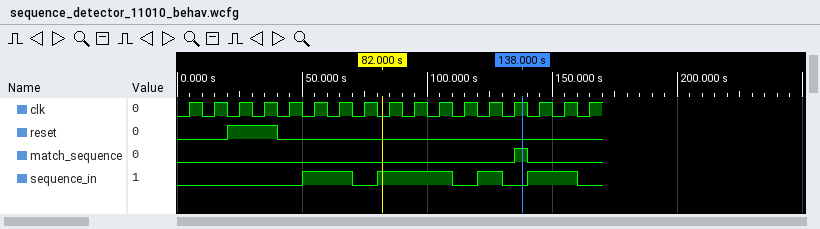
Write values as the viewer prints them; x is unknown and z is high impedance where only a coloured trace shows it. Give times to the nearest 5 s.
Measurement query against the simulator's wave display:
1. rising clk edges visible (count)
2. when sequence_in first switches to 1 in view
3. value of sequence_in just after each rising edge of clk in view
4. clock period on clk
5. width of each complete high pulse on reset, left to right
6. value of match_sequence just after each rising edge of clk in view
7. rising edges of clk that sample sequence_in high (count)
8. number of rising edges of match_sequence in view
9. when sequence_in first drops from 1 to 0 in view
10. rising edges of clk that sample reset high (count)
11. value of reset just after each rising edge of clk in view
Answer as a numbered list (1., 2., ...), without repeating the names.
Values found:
1. 17
2. 50 s
3. 0 0 0 0 0 1 1 0 1 1 1 0 1 0 1 1 0
4. 10 s
5. 20 s
6. 0 0 0 0 0 0 0 0 0 0 0 0 0 1 0 0 0
7. 8
8. 1
9. 70 s
10. 2
11. 0 0 1 1 0 0 0 0 0 0 0 0 0 0 0 0 0
